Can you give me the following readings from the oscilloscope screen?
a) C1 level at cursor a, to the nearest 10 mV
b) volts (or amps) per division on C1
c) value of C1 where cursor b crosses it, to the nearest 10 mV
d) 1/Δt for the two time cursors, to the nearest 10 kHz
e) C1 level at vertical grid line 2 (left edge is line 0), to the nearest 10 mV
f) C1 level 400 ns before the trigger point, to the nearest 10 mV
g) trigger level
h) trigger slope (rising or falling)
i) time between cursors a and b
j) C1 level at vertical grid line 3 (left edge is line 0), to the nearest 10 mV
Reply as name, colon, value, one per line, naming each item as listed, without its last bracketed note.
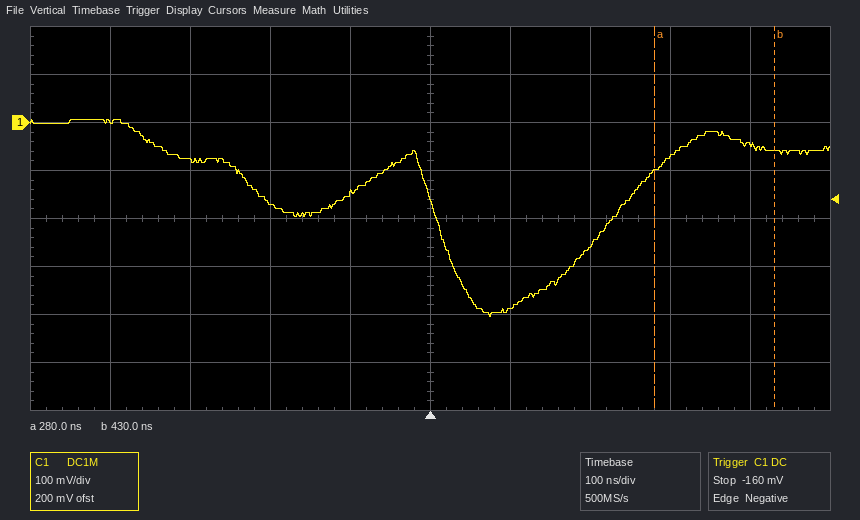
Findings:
C1 level at cursor a, to the nearest 10 mV: -100 mV
volts (or amps) per division on C1: 100 mV
value of C1 where cursor b crosses it, to the nearest 10 mV: -60 mV
1/Δt for the two time cursors, to the nearest 10 kHz: 6.67 MHz
C1 level at vertical grid line 2 (left edge is line 0), to the nearest 10 mV: -80 mV
C1 level 400 ns before the trigger point, to the nearest 10 mV: 0 mV
trigger level: -160 mV
trigger slope: falling
time between cursors a and b: 150 ns
C1 level at vertical grid line 3 (left edge is line 0), to the nearest 10 mV: -170 mV
